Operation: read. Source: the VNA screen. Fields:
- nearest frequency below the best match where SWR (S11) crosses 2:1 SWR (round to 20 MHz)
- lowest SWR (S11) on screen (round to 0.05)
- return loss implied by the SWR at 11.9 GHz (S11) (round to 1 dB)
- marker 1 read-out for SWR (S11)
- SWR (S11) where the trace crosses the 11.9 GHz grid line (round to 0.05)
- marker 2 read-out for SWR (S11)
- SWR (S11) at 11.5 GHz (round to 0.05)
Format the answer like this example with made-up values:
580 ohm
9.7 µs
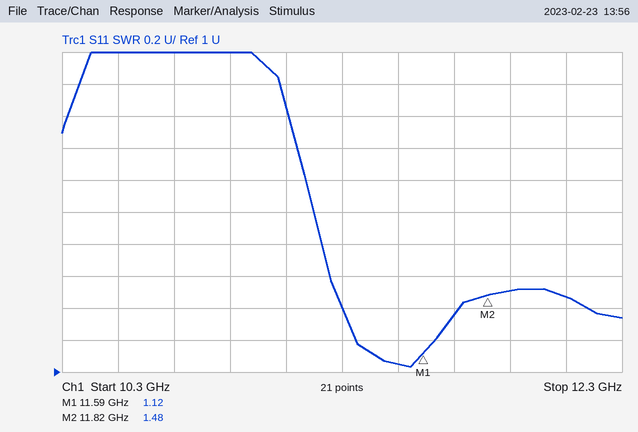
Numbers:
11.20 GHz
1.05
14 dB
1.12
1.50
1.48
1.05
